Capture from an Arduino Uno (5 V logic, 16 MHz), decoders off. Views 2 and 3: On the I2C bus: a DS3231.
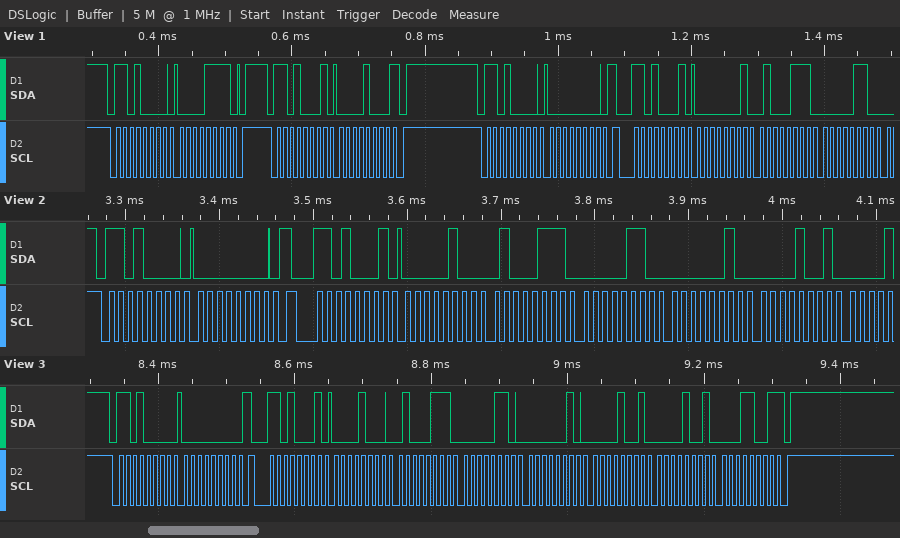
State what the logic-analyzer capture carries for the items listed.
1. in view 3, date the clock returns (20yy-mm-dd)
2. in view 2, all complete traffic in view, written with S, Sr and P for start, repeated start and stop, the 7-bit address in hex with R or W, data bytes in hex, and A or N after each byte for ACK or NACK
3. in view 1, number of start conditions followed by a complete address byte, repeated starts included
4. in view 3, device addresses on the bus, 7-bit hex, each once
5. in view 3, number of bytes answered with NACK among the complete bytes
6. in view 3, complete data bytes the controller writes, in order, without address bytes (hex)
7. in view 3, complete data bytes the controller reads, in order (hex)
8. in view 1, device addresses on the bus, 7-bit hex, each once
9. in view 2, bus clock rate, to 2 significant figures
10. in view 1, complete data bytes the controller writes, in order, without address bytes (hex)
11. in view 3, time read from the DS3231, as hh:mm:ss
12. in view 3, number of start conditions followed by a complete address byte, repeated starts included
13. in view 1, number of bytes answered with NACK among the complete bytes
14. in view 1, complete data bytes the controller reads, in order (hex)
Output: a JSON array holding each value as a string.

["2019-09-09", "S 68W A 00 A Sr 68R A 04 A 47 A 06 A 02 A 09 A", "4", "0x68", "1", "00", "08 47 06 02 09 09 19", "0x68", "100 kHz", "0F 00", "06:47:08", "2", "1", "08 01 47 06"]
